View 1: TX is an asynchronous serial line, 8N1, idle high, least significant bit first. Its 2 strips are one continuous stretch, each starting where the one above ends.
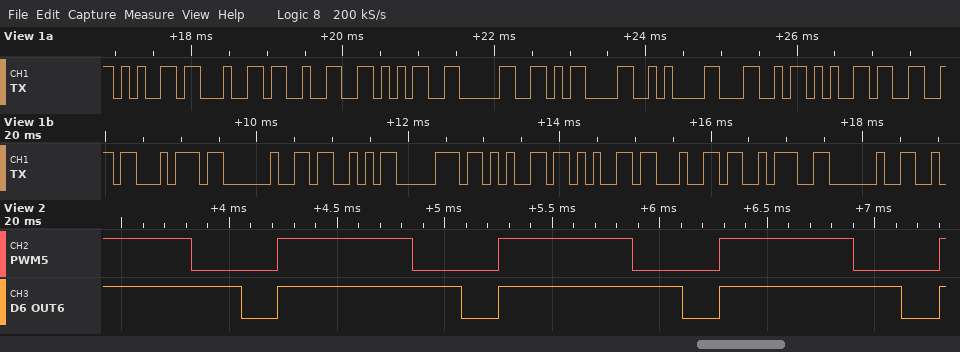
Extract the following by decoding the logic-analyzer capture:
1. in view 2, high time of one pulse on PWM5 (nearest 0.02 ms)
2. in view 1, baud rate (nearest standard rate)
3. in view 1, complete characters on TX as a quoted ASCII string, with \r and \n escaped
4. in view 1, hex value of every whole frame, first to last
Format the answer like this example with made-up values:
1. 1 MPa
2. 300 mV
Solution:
1. 0.62 ms
2. 9600 baud
3. "ed250\r\nLeft Speed: "
4. 65 64 32 35 30 0D 0A 4C 65 66 74 20 53 70 65 65 64 3A 20
